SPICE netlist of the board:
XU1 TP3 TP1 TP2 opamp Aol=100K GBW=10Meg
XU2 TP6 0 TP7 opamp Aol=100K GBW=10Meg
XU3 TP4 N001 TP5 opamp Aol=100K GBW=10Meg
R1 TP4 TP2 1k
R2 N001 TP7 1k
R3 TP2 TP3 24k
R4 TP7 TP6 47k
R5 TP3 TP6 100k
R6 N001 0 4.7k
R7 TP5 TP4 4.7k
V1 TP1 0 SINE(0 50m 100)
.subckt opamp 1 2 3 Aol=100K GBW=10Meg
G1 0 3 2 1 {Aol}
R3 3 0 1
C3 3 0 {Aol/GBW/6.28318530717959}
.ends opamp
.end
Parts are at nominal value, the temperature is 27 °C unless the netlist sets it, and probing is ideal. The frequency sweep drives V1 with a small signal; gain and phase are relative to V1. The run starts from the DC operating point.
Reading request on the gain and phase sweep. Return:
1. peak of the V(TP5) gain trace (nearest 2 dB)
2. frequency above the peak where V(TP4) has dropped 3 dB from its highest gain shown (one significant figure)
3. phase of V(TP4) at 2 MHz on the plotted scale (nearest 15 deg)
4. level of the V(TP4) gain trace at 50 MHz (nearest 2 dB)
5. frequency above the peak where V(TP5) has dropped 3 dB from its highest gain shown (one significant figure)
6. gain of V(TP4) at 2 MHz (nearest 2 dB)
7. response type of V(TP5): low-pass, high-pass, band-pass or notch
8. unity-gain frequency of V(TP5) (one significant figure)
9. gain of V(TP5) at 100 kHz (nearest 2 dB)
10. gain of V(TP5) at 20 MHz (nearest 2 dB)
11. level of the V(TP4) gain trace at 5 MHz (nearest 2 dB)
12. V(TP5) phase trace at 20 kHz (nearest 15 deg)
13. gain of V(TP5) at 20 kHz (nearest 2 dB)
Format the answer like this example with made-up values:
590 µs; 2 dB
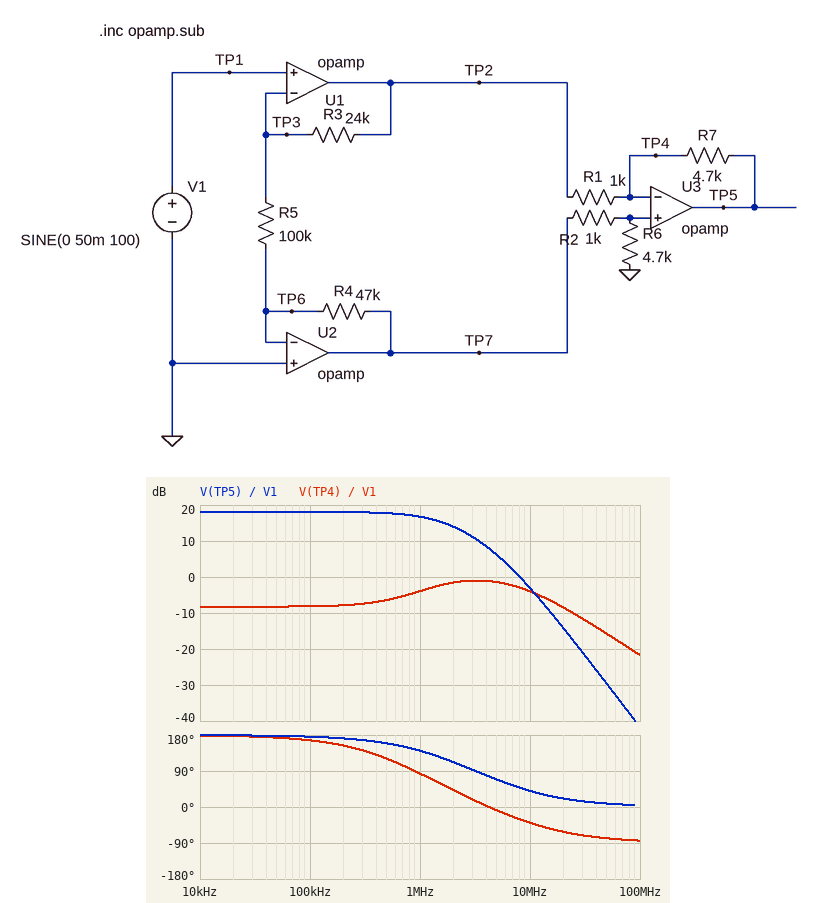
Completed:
18 dB; 10 MHz; 45 deg; -16 dB; 2 MHz; -2 dB; low-pass; 8 MHz; 18 dB; -14 dB; -2 dB; 180 deg; 18 dB
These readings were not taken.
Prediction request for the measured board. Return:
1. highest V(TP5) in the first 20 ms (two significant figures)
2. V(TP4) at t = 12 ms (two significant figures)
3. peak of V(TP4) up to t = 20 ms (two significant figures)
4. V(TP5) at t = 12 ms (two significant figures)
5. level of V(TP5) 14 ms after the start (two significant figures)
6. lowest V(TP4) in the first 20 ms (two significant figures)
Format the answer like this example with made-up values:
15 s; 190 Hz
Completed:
400 mV; -18 mV; 19 mV; -380 mV; -240 mV; -19 mV
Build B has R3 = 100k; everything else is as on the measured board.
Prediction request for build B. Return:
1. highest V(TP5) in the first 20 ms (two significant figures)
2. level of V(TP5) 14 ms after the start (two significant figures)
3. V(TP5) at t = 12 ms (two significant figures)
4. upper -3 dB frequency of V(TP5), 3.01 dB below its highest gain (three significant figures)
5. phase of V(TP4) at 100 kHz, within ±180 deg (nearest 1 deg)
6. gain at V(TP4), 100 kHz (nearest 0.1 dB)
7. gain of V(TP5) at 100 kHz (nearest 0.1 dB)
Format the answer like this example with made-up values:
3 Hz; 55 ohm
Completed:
580 mV; -340 mV; -550 mV; 1.52 MHz; 161 deg; -8.0 dB; 21.3 dB
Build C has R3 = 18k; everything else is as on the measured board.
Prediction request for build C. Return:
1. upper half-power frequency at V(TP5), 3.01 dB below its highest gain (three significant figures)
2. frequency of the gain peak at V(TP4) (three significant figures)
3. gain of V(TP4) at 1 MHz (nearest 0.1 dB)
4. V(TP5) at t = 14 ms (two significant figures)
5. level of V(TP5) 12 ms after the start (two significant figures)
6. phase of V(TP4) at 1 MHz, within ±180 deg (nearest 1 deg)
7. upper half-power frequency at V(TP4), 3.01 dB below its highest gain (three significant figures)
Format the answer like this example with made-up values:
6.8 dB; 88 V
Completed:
1.63 MHz; 3.36 MHz; -4.2 dB; -230 mV; -370 mV; 85 deg; 10.4 MHz
